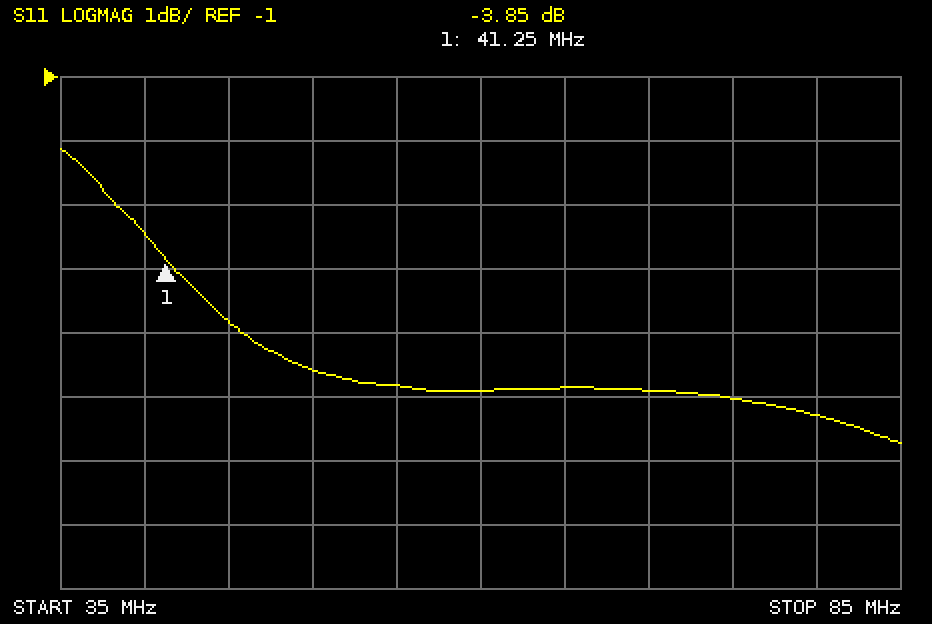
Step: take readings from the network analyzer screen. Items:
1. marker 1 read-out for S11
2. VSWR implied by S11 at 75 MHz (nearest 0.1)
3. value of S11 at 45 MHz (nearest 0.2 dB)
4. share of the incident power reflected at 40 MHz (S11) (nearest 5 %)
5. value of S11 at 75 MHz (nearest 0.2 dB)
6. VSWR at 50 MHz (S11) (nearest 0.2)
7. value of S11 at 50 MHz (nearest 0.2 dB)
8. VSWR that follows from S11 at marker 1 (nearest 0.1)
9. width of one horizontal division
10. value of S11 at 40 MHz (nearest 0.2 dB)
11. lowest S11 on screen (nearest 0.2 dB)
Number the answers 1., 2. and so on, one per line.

1. -3.85 dB
2. 3.0
3. -4.8 dB
4. 45 %
5. -6.0 dB
6. 3.2
7. -5.6 dB
8. 4.6
9. 5 MHz
10. -3.4 dB
11. -6.8 dB
